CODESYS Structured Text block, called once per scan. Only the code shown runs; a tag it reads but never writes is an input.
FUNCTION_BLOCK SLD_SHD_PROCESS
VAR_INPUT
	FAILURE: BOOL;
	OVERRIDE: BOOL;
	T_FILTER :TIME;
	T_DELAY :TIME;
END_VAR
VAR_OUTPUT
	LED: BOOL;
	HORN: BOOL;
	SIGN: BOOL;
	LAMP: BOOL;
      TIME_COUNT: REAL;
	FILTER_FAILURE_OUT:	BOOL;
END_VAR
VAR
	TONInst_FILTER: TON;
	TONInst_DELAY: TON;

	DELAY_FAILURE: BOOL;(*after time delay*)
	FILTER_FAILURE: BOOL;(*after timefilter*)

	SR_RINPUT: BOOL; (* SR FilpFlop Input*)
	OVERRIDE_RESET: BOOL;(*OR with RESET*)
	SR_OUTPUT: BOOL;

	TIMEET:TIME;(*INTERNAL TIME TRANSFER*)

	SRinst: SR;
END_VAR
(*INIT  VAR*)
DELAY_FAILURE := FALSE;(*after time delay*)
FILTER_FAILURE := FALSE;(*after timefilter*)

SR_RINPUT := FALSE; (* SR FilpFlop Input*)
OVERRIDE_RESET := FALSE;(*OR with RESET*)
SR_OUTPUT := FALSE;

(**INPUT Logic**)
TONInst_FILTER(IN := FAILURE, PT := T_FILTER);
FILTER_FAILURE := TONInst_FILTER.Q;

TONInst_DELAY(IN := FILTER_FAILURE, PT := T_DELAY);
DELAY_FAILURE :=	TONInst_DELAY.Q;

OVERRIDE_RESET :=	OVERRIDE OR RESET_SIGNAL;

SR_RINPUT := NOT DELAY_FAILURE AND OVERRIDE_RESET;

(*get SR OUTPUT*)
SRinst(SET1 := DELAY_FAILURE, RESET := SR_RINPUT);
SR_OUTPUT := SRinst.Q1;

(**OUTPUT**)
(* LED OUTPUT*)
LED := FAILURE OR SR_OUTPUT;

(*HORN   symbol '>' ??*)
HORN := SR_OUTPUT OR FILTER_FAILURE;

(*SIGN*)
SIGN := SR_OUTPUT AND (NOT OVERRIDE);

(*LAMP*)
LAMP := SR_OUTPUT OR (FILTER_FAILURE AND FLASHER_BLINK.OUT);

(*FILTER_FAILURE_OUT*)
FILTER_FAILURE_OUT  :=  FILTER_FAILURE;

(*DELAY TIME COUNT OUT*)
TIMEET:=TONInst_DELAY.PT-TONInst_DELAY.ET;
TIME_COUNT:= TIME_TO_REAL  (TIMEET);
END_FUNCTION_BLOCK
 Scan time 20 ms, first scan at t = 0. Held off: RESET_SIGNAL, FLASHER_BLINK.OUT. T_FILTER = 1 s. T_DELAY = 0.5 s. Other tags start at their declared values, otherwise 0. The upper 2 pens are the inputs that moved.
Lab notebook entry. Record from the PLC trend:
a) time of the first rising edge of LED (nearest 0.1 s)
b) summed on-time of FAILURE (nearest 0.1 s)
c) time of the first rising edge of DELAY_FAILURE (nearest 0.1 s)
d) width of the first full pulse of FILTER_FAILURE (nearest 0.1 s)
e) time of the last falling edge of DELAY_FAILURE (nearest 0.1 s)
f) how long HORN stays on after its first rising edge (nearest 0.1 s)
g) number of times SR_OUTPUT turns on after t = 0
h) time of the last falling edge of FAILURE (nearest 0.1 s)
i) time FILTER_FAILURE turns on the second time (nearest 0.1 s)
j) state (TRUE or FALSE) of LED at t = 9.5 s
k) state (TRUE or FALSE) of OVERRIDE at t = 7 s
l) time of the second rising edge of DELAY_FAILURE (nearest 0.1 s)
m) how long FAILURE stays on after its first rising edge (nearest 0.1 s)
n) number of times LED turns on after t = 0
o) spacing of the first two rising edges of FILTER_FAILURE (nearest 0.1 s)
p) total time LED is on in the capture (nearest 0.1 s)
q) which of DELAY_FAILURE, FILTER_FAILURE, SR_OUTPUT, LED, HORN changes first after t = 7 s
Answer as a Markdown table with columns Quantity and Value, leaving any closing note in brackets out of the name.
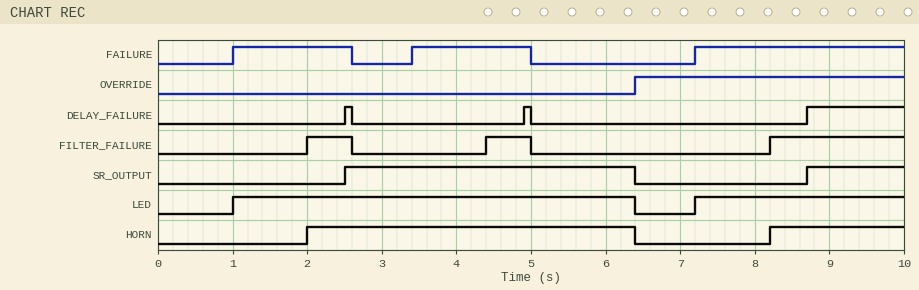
| Quantity | Value |
|---|---|
| time of the first rising edge of LED | 1.0 s |
| summed on-time of FAILURE | 6.0 s |
| time of the first rising edge of DELAY_FAILURE | 2.5 s |
| width of the first full pulse of FILTER_FAILURE | 0.6 s |
| time of the last falling edge of DELAY_FAILURE | 5.0 s |
| how long HORN stays on after its first rising edge | 4.4 s |
| number of times SR_OUTPUT turns on after t = 0 | 2 |
| time of the last falling edge of FAILURE | 5.0 s |
| time FILTER_FAILURE turns on the second time | 4.4 s |
| state (TRUE or FALSE) of LED at t = 9.5 s | TRUE |
| state (TRUE or FALSE) of OVERRIDE at t = 7 s | TRUE |
| time of the second rising edge of DELAY_FAILURE | 4.9 s |
| how long FAILURE stays on after its first rising edge | 1.6 s |
| number of times LED turns on after t = 0 | 2 |
| spacing of the first two rising edges of FILTER_FAILURE | 2.4 s |
| total time LED is on in the capture | 8.2 s |
| which of DELAY_FAILURE, FILTER_FAILURE, SR_OUTPUT, LED, HORN changes first after t = 7 s | LED |
